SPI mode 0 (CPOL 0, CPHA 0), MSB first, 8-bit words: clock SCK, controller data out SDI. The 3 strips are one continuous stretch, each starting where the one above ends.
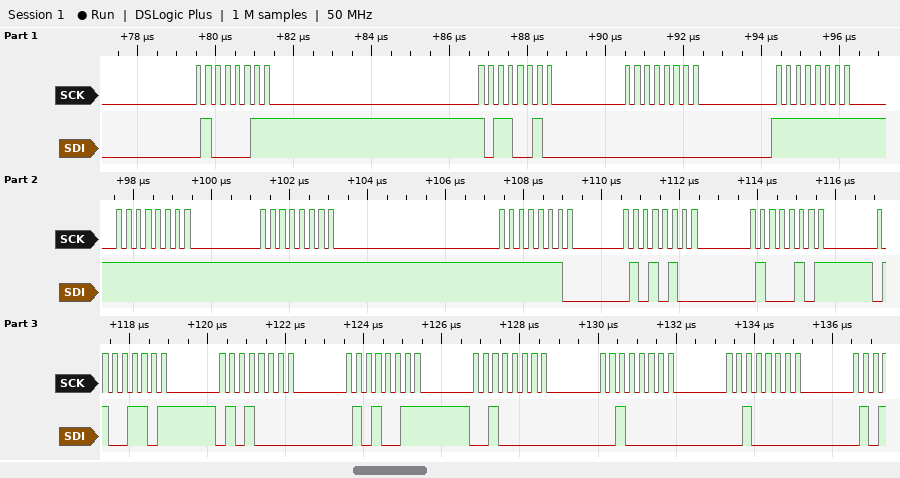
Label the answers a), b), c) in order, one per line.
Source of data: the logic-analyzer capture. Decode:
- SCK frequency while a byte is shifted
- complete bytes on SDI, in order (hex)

a) 4 MHz
b) 43 B2 00 FF FF FF FE 54 45 4D 50 53 20 20 20
